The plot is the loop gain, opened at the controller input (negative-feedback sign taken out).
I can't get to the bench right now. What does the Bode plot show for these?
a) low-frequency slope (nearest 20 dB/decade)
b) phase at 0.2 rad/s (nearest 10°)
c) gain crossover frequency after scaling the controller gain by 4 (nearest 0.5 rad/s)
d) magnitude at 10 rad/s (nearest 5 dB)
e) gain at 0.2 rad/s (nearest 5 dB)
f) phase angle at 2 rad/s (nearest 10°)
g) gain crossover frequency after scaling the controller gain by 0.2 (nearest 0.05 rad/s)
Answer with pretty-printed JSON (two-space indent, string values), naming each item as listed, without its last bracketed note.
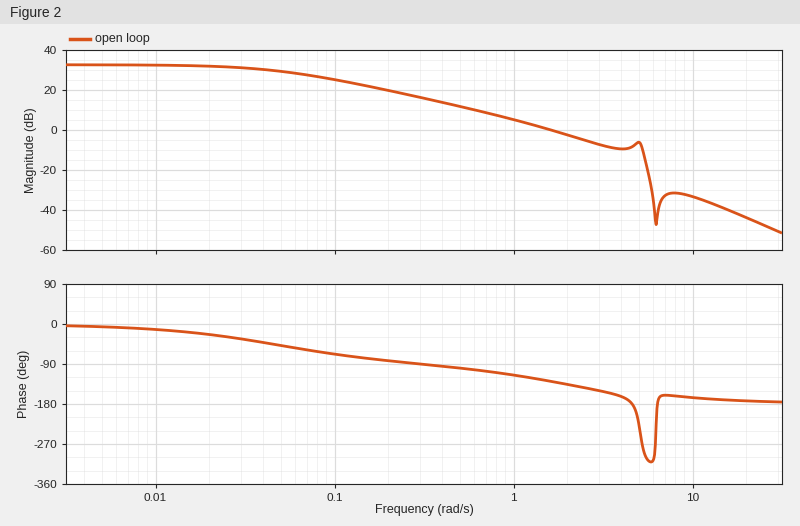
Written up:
{
  "low-frequency slope": "0 dB/decade",
  "phase at 0.2 rad/s": "-80°",
  "gain crossover frequency after scaling the controller gain by 4": "5.5 rad/s",
  "magnitude at 10 rad/s": "-35 dB",
  "gain at 0.2 rad/s": "20 dB",
  "phase angle at 2 rad/s": "-140°",
  "gain crossover frequency after scaling the controller gain by 0.2": "0.40 rad/s"
}
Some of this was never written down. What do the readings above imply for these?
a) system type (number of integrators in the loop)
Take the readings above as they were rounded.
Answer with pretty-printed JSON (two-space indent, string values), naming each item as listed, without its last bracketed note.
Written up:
{
  "system type": "0"
}
